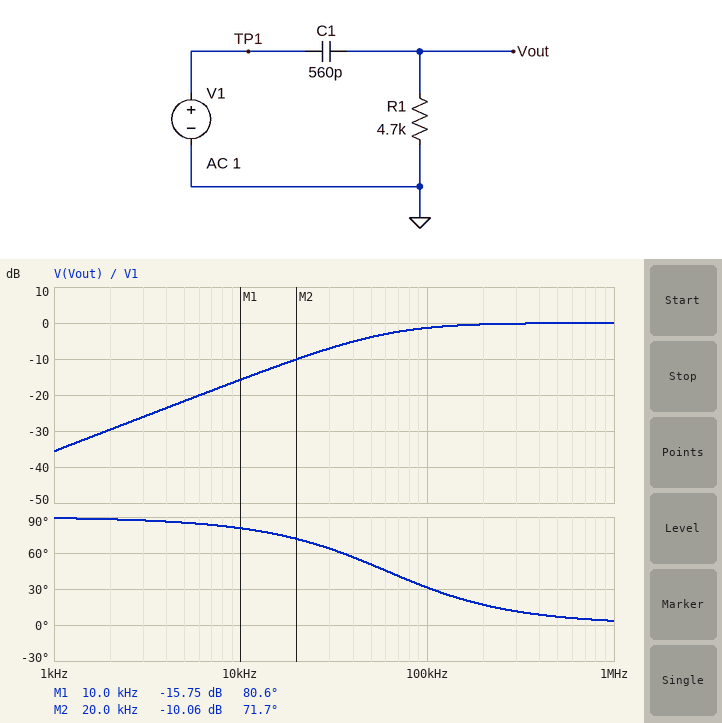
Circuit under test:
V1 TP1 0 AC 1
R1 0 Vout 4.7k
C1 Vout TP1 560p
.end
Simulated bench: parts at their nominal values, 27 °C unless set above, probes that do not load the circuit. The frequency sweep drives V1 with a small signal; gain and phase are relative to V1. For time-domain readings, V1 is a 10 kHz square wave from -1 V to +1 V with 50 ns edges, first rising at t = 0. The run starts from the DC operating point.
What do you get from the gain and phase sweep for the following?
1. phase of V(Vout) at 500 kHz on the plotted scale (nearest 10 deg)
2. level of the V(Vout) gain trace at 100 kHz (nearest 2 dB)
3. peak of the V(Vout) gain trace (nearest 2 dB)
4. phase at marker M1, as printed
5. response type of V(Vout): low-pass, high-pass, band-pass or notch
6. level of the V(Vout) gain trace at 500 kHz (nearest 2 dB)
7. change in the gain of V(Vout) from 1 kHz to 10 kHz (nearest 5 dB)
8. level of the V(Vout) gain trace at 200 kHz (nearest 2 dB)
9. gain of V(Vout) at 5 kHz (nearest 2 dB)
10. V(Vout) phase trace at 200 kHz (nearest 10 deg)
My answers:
10 deg
-2 dB
0 dB
80.6 deg
high-pass
0 dB
20 dB
0 dB
-22 dB
20 deg
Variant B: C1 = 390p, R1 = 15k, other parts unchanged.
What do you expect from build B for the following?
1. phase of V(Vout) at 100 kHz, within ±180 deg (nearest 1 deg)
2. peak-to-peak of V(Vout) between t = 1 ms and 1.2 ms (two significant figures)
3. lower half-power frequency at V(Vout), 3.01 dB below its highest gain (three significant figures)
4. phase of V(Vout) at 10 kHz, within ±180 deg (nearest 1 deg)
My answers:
15 deg
4.0 V
27.2 kHz
70 deg
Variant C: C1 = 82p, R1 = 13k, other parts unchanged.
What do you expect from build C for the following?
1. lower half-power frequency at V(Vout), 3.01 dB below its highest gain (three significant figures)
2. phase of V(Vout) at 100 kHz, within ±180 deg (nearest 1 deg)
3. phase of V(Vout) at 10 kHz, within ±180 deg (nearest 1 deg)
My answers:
149 kHz
56 deg
86 deg
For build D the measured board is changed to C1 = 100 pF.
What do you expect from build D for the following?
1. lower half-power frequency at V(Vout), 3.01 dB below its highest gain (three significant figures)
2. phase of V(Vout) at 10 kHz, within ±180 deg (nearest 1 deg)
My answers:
339 kHz
88 deg
